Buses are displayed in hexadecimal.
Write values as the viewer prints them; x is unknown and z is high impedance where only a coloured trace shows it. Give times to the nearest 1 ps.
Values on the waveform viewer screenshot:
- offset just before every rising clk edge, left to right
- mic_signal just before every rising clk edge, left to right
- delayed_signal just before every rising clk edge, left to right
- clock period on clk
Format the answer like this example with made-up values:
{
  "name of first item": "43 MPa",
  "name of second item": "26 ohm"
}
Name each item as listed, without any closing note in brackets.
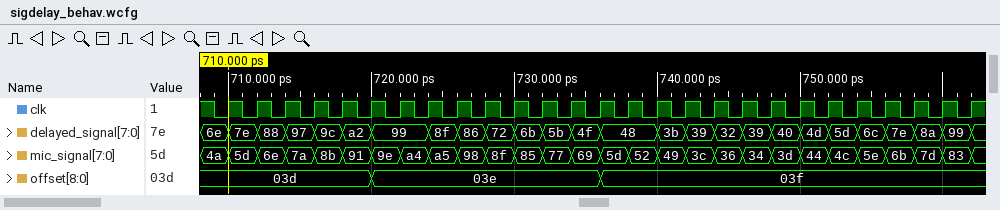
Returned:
{
  "offset just before every rising clk edge, left to right": "03d, 03d, 03d, 03d, 03d, 03d, 03e, 03e, 03e, 03e, 03e, 03e, 03e, 03e, 03f, 03f, 03f, 03f, 03f, 03f, 03f, 03f, 03f, 03f, 03f, 03f, 03f",
  "mic_signal just before every rising clk edge, left to right": "4a, 5d, 6e, 7a, 8b, 91, 9e, a4, a5, 98, 8f, 85, 77, 69, 5d, 52, 49, 3c, 36, 34, 3d, 44, 4c, 5e, 6b, 7d, 83",
  "delayed_signal just before every rising clk edge, left to right": "6e, 7e, 88, 97, 9c, a2, 99, 99, 8f, 86, 72, 6b, 5b, 4f, 48, 48, 3b, 39, 32, 39, 40, 4d, 5d, 6c, 7e, 8a, 99",
  "clock period on clk": "2 ps"
}
